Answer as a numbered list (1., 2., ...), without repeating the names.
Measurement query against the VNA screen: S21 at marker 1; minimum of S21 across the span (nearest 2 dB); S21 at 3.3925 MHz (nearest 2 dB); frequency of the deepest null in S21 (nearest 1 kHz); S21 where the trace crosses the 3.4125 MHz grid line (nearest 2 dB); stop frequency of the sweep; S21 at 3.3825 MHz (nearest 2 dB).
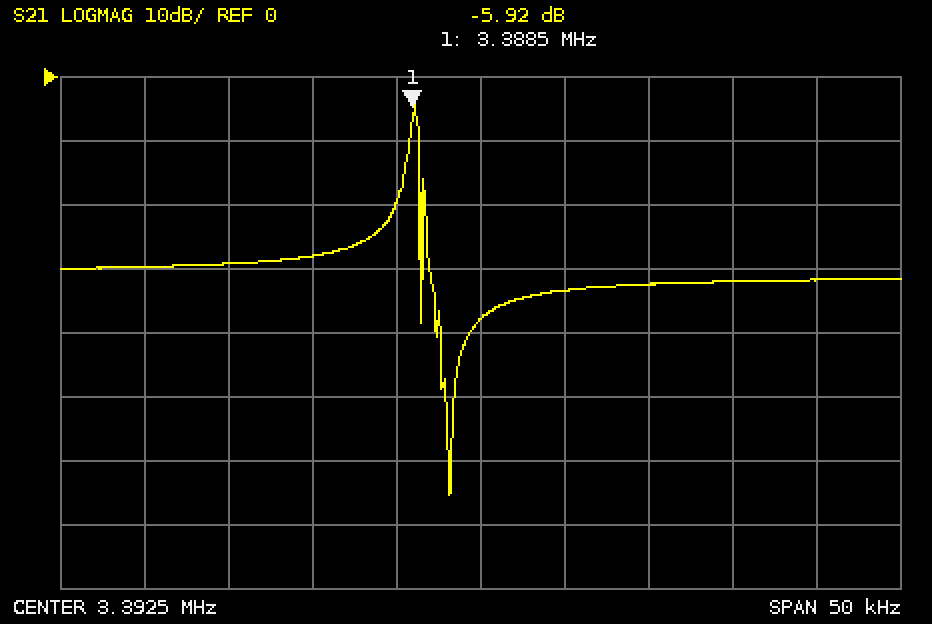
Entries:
1. -5.92 dB
2. -66 dB
3. -38 dB
4. 3.391 MHz
5. -32 dB
6. 3.4175 MHz
7. -28 dB
